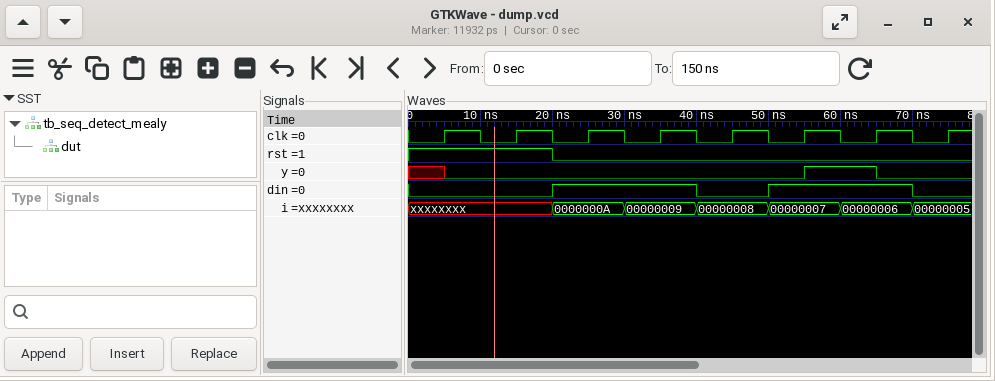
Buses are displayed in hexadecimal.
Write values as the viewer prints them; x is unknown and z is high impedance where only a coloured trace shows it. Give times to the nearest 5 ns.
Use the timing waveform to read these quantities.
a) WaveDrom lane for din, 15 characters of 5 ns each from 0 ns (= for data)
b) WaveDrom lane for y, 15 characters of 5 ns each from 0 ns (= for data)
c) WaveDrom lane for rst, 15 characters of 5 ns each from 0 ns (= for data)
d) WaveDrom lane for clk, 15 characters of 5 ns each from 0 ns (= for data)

{name: 'din', wave: '0...1...0.1...0'}
{name: 'y', wave: 'x0.........1.0.'}
{name: 'rst', wave: '1...0..........'}
{name: 'clk', wave: '010101010101010'}
